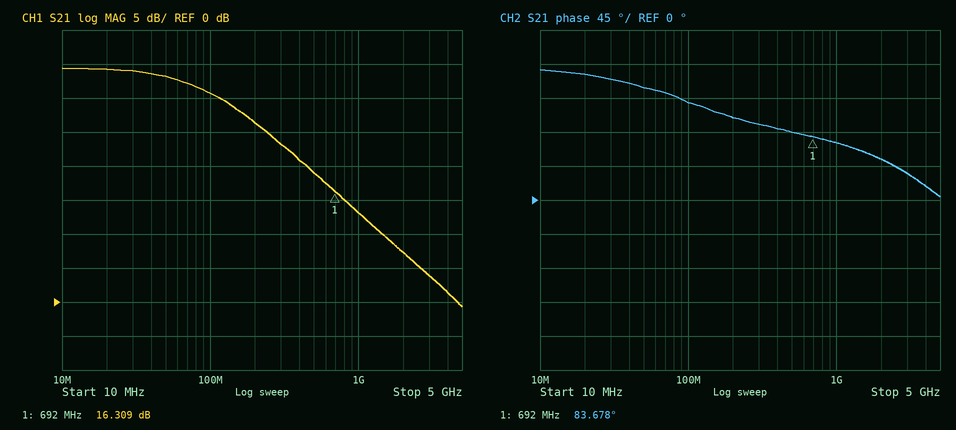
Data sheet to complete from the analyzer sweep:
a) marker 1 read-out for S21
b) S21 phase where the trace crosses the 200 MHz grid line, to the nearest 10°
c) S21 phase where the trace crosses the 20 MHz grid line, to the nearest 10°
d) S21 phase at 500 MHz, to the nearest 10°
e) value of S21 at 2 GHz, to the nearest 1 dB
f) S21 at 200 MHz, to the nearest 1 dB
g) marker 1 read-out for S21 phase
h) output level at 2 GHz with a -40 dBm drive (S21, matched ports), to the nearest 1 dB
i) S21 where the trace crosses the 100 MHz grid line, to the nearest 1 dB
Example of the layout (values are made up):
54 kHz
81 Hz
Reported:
16.309 dB
110°
170°
90°
7 dB
26 dB
83.678°
-33 dBm
31 dB
